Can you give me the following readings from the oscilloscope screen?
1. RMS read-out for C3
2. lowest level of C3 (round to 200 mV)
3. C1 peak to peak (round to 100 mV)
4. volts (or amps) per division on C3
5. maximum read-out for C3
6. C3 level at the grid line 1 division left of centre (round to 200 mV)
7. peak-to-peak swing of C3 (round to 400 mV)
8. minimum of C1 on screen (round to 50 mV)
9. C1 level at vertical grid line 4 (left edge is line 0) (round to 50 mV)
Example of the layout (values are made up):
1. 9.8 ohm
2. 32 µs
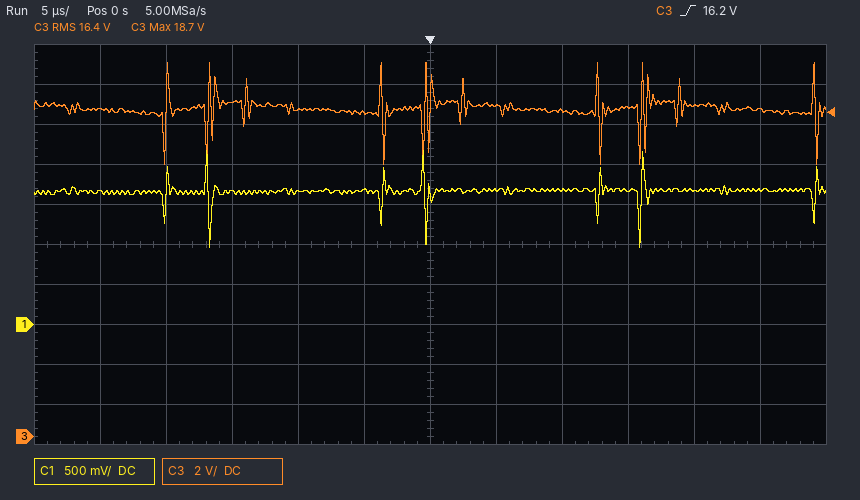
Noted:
1. 16.4 V
2. 13.6 V
3. 1.20 V
4. 2 V
5. 18.7 V
6. 16.2 V
7. 5.2 V
8. 950 mV
9. 1.65 V
